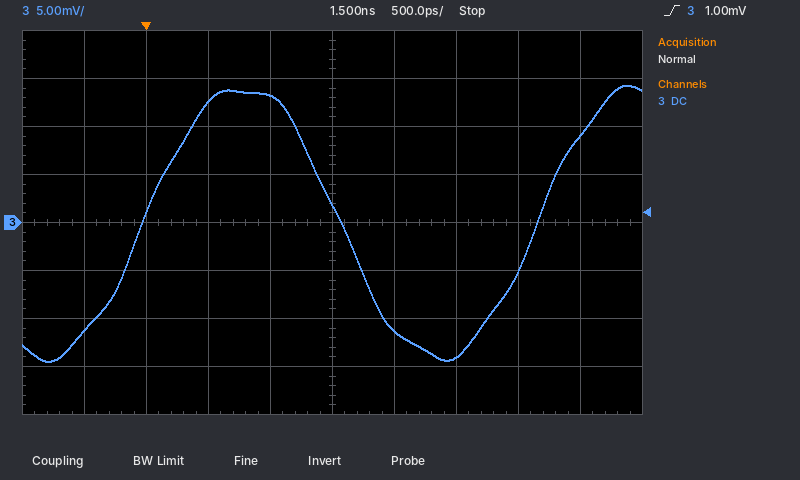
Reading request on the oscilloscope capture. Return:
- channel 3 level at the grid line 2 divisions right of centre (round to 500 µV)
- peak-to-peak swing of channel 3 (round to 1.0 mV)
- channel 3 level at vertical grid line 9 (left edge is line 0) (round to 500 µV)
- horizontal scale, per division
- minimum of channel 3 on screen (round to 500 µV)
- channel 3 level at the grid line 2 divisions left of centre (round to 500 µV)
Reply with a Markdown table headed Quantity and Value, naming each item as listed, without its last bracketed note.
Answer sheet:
| Quantity | Value |
|---|---|
| channel 3 level at the grid line 2 divisions right of centre | -14.0 mV |
| peak-to-peak swing of channel 3 | 29.0 mV |
| channel 3 level at vertical grid line 9 (left edge is line 0) | 9.0 mV |
| horizontal scale, per division | 500 ps |
| minimum of channel 3 on screen | -14.5 mV |
| channel 3 level at the grid line 2 divisions left of centre | 12.5 mV |
